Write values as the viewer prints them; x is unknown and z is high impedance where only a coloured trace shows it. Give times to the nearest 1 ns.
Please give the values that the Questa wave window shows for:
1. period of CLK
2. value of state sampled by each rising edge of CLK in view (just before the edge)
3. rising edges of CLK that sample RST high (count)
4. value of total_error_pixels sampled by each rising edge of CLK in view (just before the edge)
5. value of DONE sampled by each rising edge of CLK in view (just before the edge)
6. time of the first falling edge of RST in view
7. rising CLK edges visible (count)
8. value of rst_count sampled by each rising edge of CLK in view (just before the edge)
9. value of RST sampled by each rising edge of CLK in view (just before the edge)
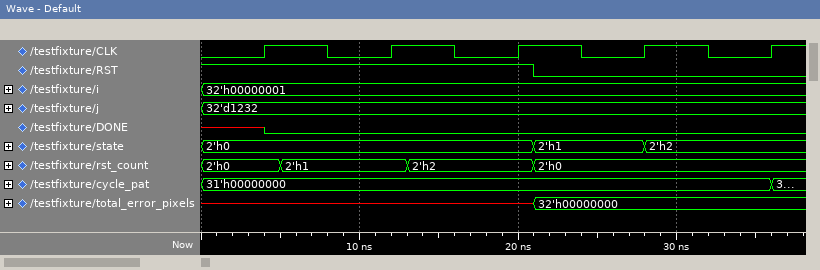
8 ns
2'h0, 2'h0, 2'h0, 2'h1, 2'h2
3
x, x, x, 32'h00000000, 32'h00000000
x 0 0 0 0
21 ns
5
2'h0, 2'h1, 2'h2, 2'h0, 2'h0
1 1 1 0 0
